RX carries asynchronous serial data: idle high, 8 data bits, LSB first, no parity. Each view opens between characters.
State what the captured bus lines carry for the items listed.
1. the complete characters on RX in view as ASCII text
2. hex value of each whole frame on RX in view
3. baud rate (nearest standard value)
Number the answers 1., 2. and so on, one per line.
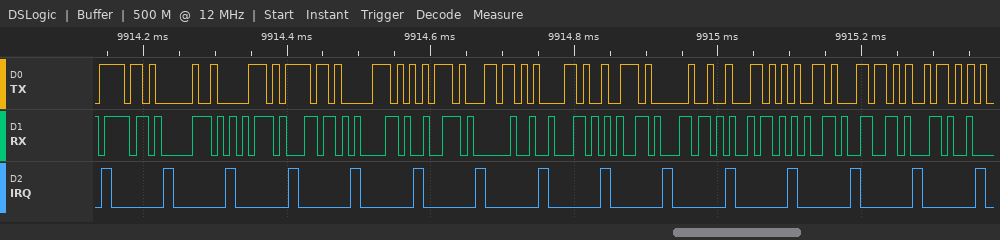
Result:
1. "opular belief,"
2. 6F, 70, 75, 6C, 61, 72, 20, 62, 65, 6C, 69, 65, 66, 2C
3. 115200 baud
